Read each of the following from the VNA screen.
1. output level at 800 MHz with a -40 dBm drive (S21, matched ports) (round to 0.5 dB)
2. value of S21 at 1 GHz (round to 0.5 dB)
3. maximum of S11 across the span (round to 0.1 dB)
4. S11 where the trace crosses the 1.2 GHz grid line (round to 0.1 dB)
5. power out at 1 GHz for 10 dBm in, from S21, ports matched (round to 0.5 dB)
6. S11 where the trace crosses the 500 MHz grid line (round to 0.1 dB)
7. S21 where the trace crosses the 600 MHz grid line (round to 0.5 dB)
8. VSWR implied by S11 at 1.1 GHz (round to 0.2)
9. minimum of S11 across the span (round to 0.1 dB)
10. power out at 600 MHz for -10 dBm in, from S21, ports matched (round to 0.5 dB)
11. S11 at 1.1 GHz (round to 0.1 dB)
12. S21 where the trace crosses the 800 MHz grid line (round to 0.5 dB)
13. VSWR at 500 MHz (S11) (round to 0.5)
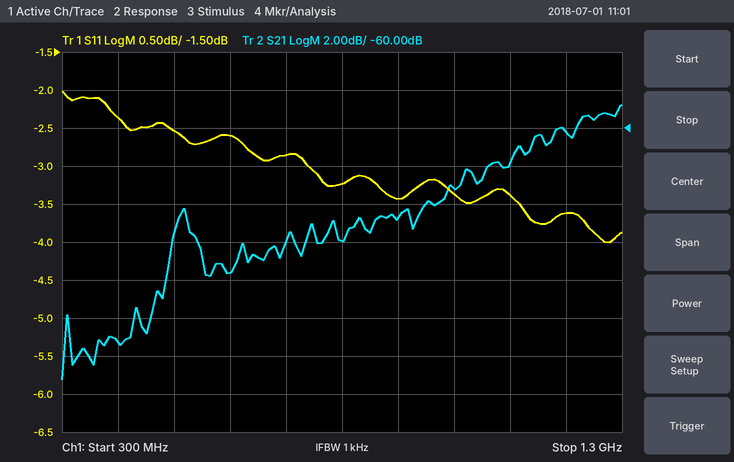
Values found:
-106.0 dBm
-63.0 dB
-2.0 dB
-3.6 dB
-53.0 dBm
-2.5 dB
-67.5 dB
5.2
-4.0 dB
-77.5 dBm
-3.4 dB
-66.0 dB
7.0
